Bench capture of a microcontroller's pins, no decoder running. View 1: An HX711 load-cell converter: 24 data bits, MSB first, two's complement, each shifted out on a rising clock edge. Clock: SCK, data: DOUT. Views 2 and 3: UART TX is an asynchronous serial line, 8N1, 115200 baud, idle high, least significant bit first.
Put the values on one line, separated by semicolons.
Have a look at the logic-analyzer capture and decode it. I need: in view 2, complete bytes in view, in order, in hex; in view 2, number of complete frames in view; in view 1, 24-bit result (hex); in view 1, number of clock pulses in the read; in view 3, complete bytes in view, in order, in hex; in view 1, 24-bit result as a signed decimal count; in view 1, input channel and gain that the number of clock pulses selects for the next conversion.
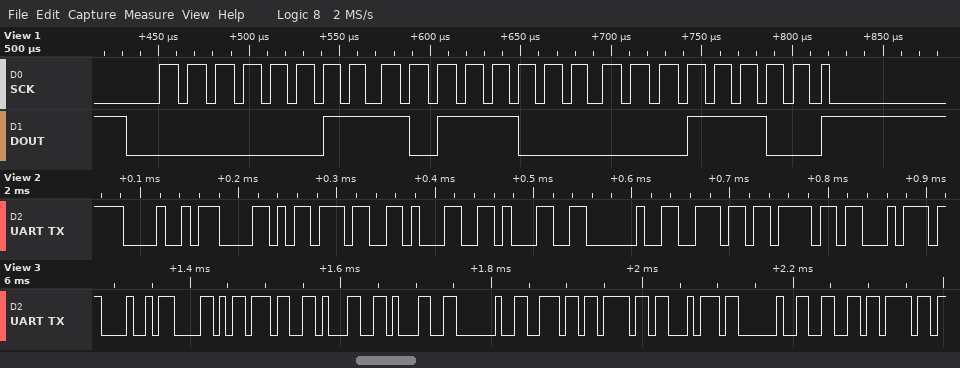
48 58 37 31 31 20 6E 6F 74; 9; 0x03B81C; 25; 0x48 0x58 0x37 0x31 0x31 0x20 0x6E 0x6F 0x74 0x20 0x66 0x6F; 243740; channel A, gain 128
